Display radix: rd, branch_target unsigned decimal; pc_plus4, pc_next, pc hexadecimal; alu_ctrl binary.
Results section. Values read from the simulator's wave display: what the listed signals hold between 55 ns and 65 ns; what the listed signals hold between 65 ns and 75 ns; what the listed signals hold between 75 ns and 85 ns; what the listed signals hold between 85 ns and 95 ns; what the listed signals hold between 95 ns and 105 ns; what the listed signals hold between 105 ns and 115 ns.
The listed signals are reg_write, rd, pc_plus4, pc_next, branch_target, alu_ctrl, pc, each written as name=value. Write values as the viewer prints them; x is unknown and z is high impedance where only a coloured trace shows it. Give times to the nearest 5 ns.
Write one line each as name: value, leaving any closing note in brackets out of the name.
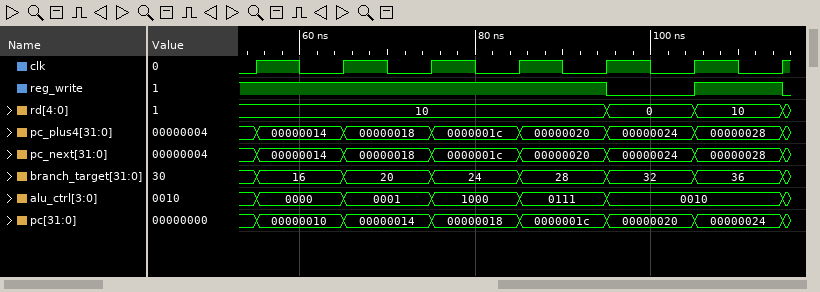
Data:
what the listed signals hold between 55 ns and 65 ns: reg_write=1, rd=10, pc_plus4=00000014, pc_next=00000014, branch_target=16, alu_ctrl=0000, pc=00000010
what the listed signals hold between 65 ns and 75 ns: reg_write=1, rd=10, pc_plus4=00000018, pc_next=00000018, branch_target=20, alu_ctrl=0001, pc=00000014
what the listed signals hold between 75 ns and 85 ns: reg_write=1, rd=10, pc_plus4=0000001c, pc_next=0000001c, branch_target=24, alu_ctrl=1000, pc=00000018
what the listed signals hold between 85 ns and 95 ns: reg_write=1, rd=10, pc_plus4=00000020, pc_next=00000020, branch_target=28, alu_ctrl=0111, pc=0000001c
what the listed signals hold between 95 ns and 105 ns: reg_write=0, rd=0, pc_plus4=00000024, pc_next=00000024, branch_target=32, alu_ctrl=0010, pc=00000020
what the listed signals hold between 105 ns and 115 ns: reg_write=1, rd=10, pc_plus4=00000028, pc_next=00000028, branch_target=36, alu_ctrl=0010, pc=00000024
